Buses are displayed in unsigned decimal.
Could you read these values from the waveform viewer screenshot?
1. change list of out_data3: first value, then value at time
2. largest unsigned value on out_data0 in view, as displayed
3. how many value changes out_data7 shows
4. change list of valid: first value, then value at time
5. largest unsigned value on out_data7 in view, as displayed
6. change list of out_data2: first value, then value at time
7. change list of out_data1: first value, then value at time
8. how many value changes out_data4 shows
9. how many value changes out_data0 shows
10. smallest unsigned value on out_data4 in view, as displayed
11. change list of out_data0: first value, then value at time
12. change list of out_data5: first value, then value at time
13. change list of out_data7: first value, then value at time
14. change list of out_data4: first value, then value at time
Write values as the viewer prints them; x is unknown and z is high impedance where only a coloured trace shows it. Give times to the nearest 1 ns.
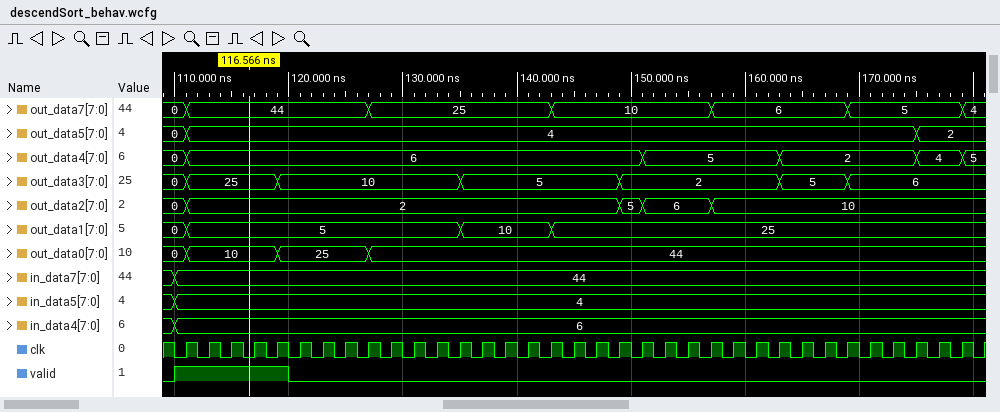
0, 25 at 111 ns, 10 at 119 ns, 5 at 135 ns, 2 at 149 ns, 5 at 163 ns, 6 at 169 ns
44
6
0, 1 at 110 ns, 0 at 120 ns
44
0, 2 at 111 ns, 5 at 149 ns, 6 at 151 ns, 10 at 157 ns
0, 5 at 111 ns, 10 at 135 ns, 25 at 143 ns
5
3
0
0, 10 at 111 ns, 25 at 119 ns, 44 at 127 ns
0, 4 at 111 ns, 2 at 175 ns
0, 44 at 111 ns, 25 at 127 ns, 10 at 143 ns, 6 at 157 ns, 5 at 169 ns, 4 at 179 ns
0, 6 at 111 ns, 5 at 151 ns, 2 at 163 ns, 4 at 175 ns, 5 at 179 ns
